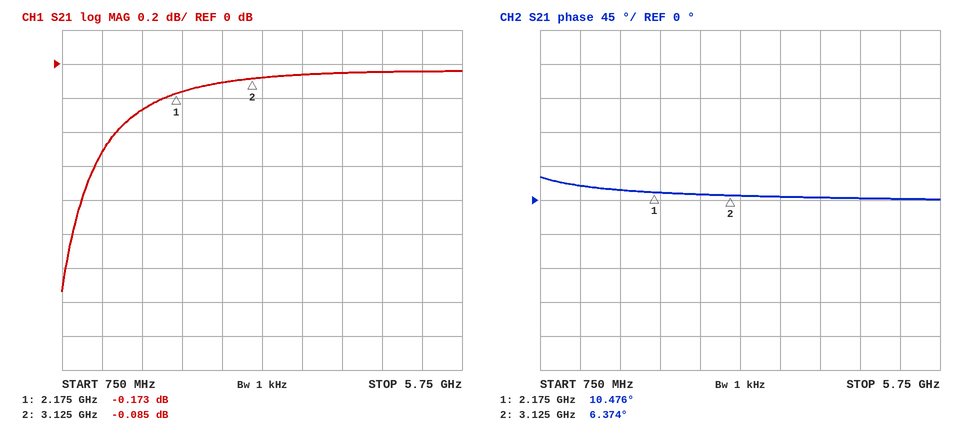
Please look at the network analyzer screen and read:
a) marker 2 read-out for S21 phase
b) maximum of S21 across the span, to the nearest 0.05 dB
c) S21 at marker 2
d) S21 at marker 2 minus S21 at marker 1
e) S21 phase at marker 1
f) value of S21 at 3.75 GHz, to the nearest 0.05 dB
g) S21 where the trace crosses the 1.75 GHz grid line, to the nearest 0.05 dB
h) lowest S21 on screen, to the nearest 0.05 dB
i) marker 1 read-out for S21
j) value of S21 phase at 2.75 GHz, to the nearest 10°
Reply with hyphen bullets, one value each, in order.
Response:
- 6.374°
- -0.05 dB
- -0.085 dB
- 0.088 dB
- 10.476°
- -0.05 dB
- -0.25 dB
- -1.35 dB
- -0.173 dB
- 10°
